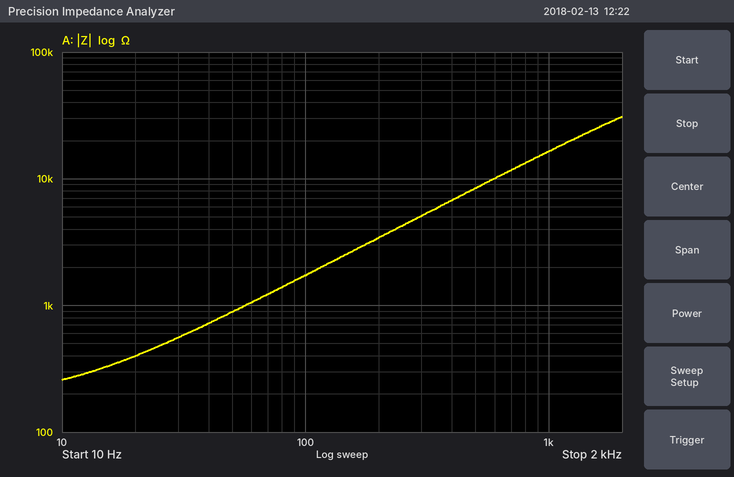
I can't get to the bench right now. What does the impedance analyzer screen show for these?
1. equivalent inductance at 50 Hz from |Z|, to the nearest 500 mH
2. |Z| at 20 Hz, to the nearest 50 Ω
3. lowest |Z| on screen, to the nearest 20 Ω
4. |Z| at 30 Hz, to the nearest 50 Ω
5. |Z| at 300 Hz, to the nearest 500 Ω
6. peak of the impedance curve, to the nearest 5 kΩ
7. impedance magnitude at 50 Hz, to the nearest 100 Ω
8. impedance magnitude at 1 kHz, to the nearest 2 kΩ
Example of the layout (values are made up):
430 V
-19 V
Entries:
3.0 H
400 Ω
260 Ω
550 Ω
5.0 kΩ
30 kΩ
900 Ω
16 kΩ
